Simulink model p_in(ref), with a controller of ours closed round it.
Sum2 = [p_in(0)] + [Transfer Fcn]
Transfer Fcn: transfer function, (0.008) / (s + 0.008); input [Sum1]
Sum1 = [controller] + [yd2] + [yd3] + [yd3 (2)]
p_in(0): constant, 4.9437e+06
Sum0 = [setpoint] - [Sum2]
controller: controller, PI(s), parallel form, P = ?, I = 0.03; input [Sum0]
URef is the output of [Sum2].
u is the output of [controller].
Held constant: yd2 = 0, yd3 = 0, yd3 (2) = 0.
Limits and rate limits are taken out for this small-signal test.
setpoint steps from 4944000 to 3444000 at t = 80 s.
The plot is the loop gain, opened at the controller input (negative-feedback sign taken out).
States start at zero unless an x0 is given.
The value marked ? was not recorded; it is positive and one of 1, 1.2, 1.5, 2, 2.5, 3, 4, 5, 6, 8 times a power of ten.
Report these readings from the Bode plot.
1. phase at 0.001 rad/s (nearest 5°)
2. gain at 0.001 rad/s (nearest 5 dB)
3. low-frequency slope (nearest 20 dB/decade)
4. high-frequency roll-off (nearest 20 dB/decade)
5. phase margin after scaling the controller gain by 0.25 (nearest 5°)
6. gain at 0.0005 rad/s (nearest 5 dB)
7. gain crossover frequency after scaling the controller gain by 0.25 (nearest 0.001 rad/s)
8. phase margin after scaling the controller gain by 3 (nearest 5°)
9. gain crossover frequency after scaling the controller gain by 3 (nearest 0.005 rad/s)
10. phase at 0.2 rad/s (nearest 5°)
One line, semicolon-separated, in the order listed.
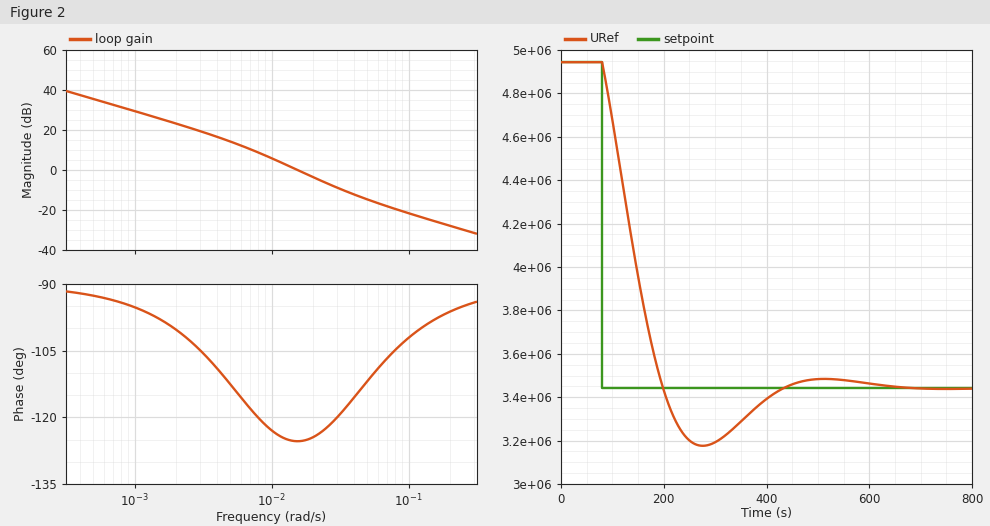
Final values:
-95°; 30 dB; -20 dB/decade; -20 dB/decade; 65°; 35 dB; 0.006 rad/s; 60°; 0.030 rad/s; -95°
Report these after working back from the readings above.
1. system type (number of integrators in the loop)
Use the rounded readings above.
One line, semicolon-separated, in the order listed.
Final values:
1
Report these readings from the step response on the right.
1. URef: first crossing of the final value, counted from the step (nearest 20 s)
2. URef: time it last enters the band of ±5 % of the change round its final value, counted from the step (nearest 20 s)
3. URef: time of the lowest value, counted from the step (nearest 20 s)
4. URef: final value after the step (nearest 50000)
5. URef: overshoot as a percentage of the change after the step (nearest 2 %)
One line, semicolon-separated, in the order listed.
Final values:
120 s; 300 s; 200 s; 3450000; 18 %
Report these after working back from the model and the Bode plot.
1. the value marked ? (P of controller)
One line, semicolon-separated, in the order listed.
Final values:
1
